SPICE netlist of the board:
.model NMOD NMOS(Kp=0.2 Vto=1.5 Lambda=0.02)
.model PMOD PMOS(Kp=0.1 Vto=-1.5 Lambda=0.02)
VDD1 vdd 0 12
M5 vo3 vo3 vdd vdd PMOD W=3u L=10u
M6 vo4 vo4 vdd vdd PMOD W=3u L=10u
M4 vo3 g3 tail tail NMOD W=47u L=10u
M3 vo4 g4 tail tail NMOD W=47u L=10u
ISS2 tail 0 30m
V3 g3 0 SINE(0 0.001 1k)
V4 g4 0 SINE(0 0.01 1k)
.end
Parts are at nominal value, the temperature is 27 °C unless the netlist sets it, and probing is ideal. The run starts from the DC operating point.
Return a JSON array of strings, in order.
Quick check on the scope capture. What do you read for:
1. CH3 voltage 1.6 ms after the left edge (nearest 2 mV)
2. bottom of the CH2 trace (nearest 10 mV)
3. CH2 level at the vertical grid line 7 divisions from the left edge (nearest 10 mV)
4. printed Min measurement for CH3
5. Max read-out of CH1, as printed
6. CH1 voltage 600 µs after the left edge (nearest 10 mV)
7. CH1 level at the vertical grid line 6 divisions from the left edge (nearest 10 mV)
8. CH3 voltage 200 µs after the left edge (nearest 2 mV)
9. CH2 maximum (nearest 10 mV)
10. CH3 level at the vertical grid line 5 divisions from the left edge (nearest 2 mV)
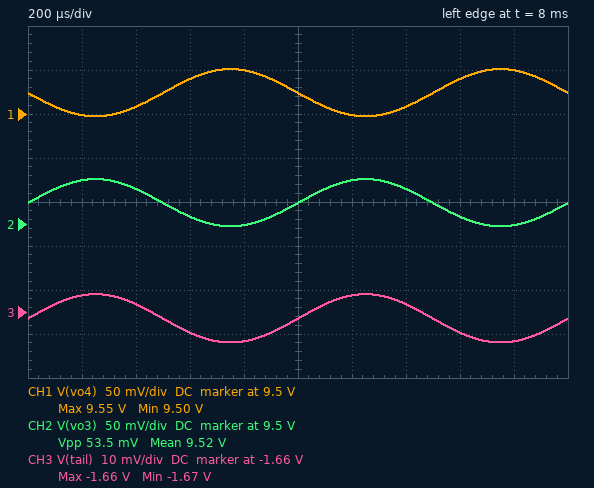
["-1.664 V", "9.50 V", "9.54 V", "-1.67 V", "9.55 V", "9.54 V", "9.50 V", "-1.656 V", "9.55 V", "-1.662 V"]
